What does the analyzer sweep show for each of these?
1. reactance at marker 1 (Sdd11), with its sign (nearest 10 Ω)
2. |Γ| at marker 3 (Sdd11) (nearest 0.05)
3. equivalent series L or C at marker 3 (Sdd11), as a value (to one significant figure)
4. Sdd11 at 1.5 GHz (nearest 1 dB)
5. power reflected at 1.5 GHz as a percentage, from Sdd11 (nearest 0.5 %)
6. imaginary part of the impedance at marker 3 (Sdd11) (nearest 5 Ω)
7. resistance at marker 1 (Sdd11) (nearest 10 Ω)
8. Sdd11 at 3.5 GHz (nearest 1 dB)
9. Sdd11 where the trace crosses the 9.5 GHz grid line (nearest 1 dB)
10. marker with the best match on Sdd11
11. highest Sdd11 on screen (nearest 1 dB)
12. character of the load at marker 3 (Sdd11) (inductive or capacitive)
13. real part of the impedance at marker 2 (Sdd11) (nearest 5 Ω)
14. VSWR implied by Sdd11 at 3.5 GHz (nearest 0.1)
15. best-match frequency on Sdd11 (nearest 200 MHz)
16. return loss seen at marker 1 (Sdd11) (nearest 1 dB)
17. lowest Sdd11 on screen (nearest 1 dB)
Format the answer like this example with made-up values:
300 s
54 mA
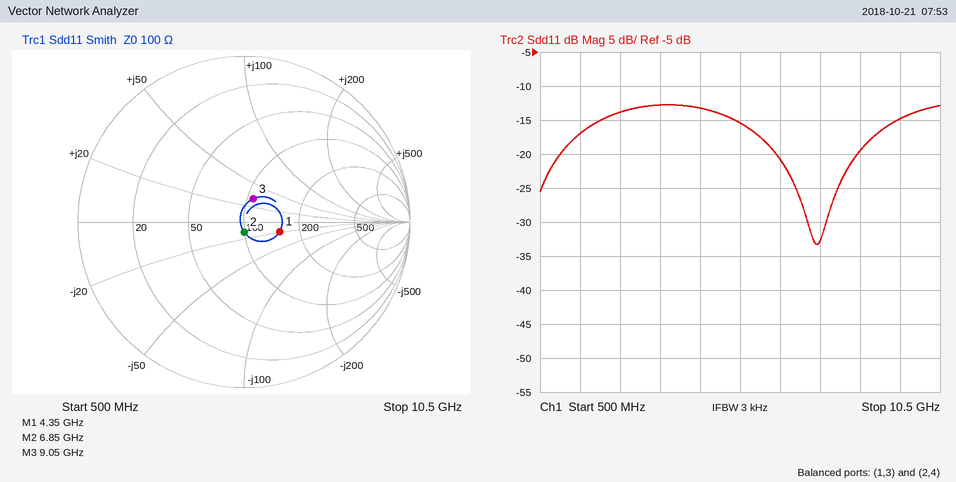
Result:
-20 Ω
0.15
500 pH
-17 dB
2.0 %
+30 Ω
150 Ω
-13 dB
-15 dB
marker 2
-13 dB
inductive
100 Ω
1.6
7.4 GHz
13 dB
-33 dB
